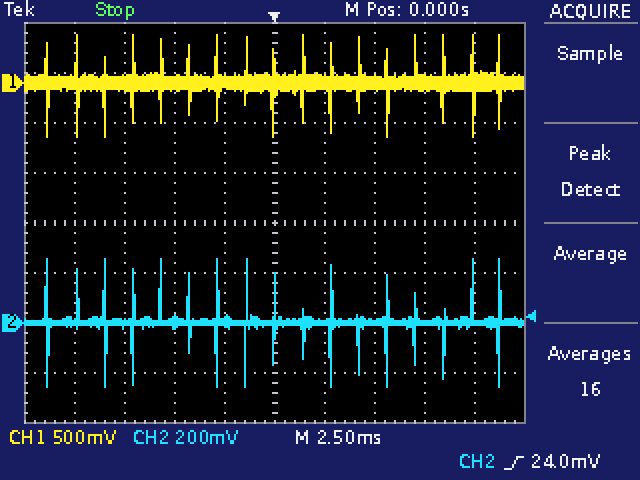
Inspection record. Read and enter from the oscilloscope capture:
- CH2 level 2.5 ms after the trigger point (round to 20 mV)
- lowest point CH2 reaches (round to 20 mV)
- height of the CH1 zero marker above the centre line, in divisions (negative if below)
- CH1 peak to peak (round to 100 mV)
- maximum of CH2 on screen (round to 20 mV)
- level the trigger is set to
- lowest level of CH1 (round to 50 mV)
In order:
0 mV
-260 mV
+2.8 div
1.00 V
260 mV
24.0 mV
-550 mV
